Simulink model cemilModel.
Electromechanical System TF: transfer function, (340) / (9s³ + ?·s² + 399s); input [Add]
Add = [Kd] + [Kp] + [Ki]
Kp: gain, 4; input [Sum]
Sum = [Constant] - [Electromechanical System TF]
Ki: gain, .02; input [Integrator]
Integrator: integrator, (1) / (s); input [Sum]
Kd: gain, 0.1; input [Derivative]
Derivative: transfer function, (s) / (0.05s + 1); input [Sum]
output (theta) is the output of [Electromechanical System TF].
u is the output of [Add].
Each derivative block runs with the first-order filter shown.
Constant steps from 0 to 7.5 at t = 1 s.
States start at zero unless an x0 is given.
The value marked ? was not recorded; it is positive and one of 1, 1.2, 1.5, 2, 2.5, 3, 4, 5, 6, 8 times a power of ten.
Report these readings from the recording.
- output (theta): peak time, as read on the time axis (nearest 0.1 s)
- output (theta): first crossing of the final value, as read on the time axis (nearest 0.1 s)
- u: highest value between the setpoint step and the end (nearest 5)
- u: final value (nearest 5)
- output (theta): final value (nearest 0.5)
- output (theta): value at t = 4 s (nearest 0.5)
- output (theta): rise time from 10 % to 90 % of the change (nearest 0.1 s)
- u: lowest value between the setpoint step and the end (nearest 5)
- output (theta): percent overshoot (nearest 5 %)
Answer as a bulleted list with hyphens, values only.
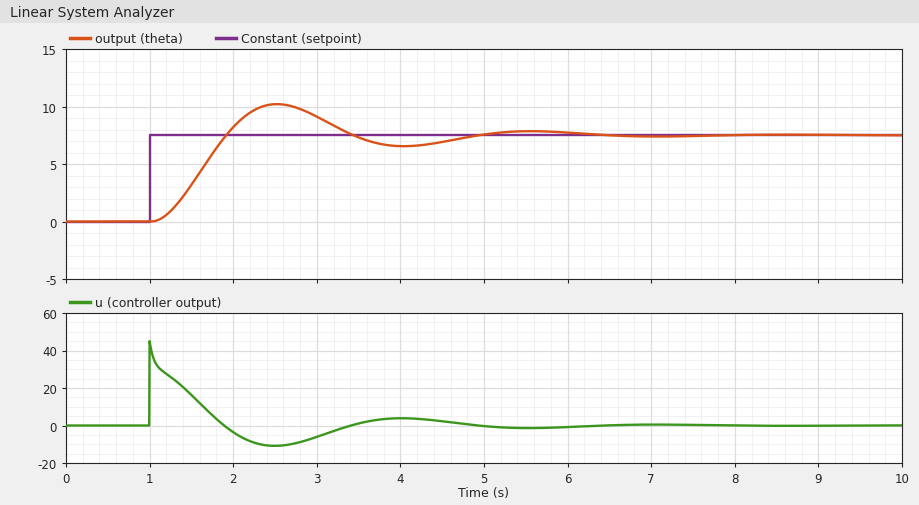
- 2.5 s
- 1.9 s
- 45
- 0
- 7.5
- 6.5
- 0.6 s
- -10
- 35 %
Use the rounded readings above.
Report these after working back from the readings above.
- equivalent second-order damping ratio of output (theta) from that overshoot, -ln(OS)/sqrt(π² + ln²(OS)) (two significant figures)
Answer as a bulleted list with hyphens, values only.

- 0.32
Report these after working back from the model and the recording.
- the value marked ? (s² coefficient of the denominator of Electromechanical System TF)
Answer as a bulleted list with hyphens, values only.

- 300
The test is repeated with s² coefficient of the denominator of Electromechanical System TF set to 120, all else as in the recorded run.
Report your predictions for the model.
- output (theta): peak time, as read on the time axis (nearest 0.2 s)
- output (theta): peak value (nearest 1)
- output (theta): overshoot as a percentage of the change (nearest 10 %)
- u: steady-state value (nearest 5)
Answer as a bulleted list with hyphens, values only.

- 2.0 s
- 9
- 20 %
- 0
